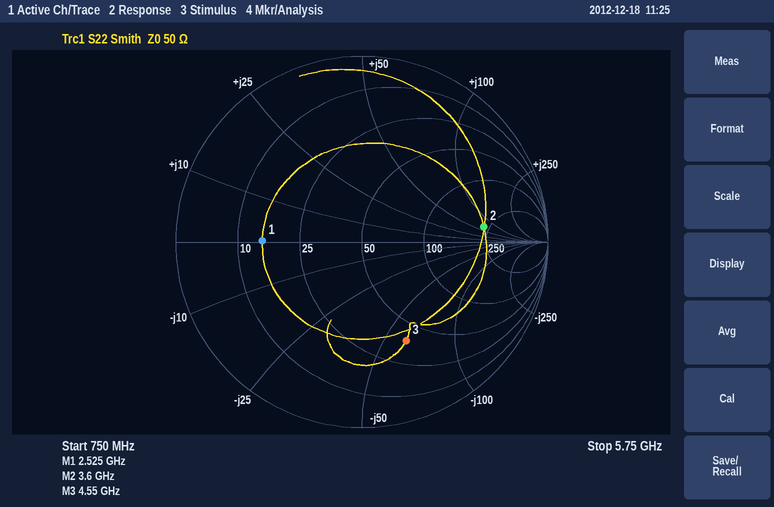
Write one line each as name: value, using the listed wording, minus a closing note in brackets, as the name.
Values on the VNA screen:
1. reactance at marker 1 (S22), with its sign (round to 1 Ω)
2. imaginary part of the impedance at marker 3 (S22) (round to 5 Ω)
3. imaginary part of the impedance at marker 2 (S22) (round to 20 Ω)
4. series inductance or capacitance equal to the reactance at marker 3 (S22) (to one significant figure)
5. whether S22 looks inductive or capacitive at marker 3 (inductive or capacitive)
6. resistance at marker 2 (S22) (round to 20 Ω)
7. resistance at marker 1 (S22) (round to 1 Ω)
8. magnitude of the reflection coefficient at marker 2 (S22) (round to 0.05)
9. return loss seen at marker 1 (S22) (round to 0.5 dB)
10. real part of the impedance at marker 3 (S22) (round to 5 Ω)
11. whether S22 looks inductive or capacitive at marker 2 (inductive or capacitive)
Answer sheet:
reactance at marker 1 (S22), with its sign: 0 Ω
imaginary part of the impedance at marker 3 (S22): -60 Ω
imaginary part of the impedance at marker 2 (S22): +60 Ω
series inductance or capacitance equal to the reactance at marker 3 (S22): 600 fF
whether S22 looks inductive or capacitive at marker 3: capacitive
resistance at marker 2 (S22): 220 Ω
resistance at marker 1 (S22): 15 Ω
magnitude of the reflection coefficient at marker 2 (S22): 0.65
return loss seen at marker 1 (S22): 5.5 dB
real part of the impedance at marker 3 (S22): 40 Ω
whether S22 looks inductive or capacitive at marker 2: inductive
